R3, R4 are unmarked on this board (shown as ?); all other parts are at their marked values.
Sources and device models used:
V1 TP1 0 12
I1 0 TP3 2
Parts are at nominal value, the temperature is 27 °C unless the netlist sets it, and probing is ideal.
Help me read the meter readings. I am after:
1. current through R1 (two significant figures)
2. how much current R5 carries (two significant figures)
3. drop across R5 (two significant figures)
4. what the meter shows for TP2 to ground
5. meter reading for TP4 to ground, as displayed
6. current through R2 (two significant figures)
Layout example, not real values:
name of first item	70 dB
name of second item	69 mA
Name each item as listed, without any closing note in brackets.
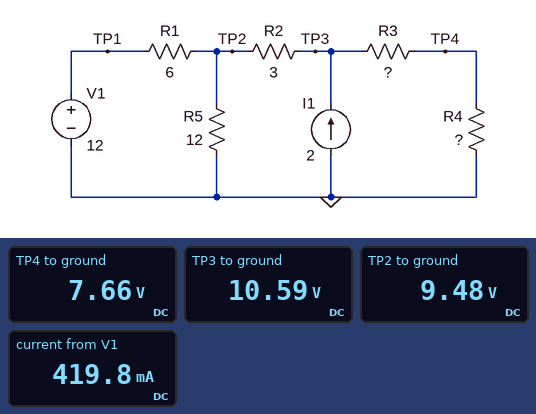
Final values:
current through R1	420 mA
how much current R5 carries	790 mA
drop across R5	9.5 V
what the meter shows for TP2 to ground	9.48 V
meter reading for TP4 to ground, as displayed	7.66 V
current through R2	370 mA
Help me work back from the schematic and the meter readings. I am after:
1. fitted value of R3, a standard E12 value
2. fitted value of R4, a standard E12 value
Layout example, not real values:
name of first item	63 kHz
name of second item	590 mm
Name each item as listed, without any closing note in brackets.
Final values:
fitted value of R3, a standard E12 value	1.8 Ω
fitted value of R4, a standard E12 value	4.7 Ω
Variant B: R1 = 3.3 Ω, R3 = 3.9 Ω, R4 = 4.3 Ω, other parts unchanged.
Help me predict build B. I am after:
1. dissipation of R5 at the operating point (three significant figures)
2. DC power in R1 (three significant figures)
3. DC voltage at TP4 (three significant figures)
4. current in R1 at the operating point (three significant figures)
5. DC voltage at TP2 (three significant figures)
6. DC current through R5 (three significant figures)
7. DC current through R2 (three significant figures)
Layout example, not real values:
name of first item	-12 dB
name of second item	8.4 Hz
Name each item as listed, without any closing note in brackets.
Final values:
dissipation of R5 at the operating point	9.58 W
DC power in R1	494 mW
DC voltage at TP4	6.42 V
current in R1 at the operating point	387 mA
DC voltage at TP2	10.7 V
DC current through R5	894 mA
DC current through R2	507 mA
